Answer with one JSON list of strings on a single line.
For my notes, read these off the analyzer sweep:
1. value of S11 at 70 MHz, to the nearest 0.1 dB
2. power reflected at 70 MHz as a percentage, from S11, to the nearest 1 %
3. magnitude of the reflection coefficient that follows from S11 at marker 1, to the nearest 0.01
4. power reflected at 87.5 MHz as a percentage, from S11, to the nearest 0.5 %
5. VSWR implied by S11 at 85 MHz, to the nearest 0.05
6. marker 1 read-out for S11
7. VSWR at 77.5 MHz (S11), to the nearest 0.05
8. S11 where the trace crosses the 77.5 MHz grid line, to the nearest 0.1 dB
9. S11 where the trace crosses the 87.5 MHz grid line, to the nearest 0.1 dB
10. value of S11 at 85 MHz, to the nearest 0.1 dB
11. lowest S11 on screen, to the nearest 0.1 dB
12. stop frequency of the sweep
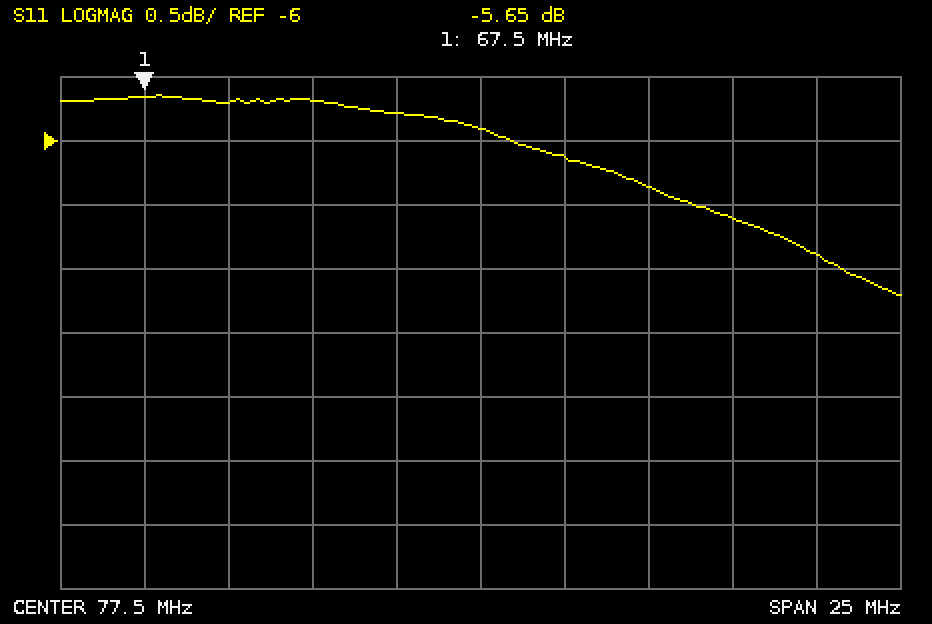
["-5.7 dB", "27 %", "0.52", "20.5 %", "2.75", "-5.65 dB", "3.05", "-5.9 dB", "-6.9 dB", "-6.6 dB", "-7.2 dB", "90 MHz"]
